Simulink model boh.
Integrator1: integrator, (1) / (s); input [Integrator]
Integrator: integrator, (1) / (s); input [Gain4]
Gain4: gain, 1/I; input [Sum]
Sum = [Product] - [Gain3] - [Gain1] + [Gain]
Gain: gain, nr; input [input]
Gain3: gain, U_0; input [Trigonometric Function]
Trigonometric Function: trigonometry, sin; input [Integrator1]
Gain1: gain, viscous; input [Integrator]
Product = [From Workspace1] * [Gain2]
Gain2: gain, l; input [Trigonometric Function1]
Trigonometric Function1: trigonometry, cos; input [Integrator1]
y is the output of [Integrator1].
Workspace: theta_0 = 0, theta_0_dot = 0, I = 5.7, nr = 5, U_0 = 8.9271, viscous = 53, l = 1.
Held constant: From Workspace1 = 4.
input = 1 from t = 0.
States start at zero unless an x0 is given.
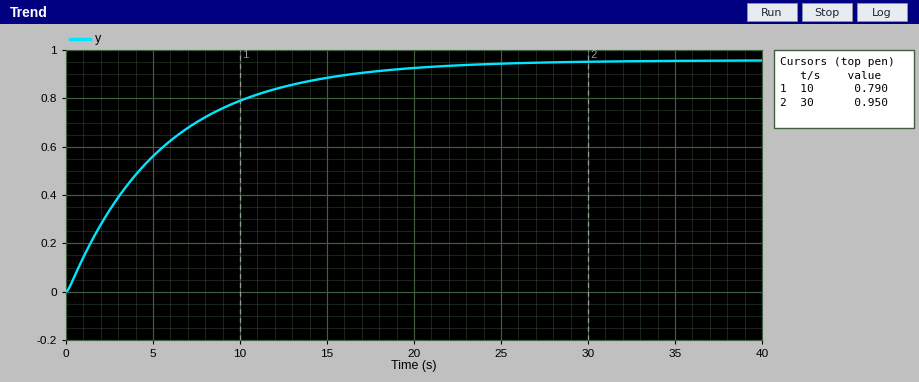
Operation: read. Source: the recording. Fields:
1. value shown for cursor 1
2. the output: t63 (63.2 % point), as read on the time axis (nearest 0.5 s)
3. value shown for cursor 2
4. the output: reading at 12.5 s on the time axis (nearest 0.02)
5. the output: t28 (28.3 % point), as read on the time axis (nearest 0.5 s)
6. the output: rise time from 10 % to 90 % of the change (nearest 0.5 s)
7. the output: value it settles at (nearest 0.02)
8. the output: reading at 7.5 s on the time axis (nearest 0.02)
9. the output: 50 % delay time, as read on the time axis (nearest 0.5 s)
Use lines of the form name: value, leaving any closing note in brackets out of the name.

value shown for cursor 1: 0.790
the output: t63 (63.2 % point), as read on the time axis: 5.5 s
value shown for cursor 2: 0.950
the output: reading at 12.5 s on the time axis: 0.84
the output: t28 (28.3 % point), as read on the time axis: 2.0 s
the output: rise time from 10 % to 90 % of the change: 12.5 s
the output: value it settles at: 0.96
the output: reading at 7.5 s on the time axis: 0.70
the output: 50 % delay time, as read on the time axis: 4.0 s
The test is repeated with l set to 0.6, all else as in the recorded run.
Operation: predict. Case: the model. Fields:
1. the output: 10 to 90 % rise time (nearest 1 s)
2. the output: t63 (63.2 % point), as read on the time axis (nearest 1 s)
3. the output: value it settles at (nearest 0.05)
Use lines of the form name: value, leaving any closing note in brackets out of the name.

the output: 10 to 90 % rise time: 14 s
the output: t63 (63.2 % point), as read on the time axis: 6 s
the output: value it settles at: 0.85
